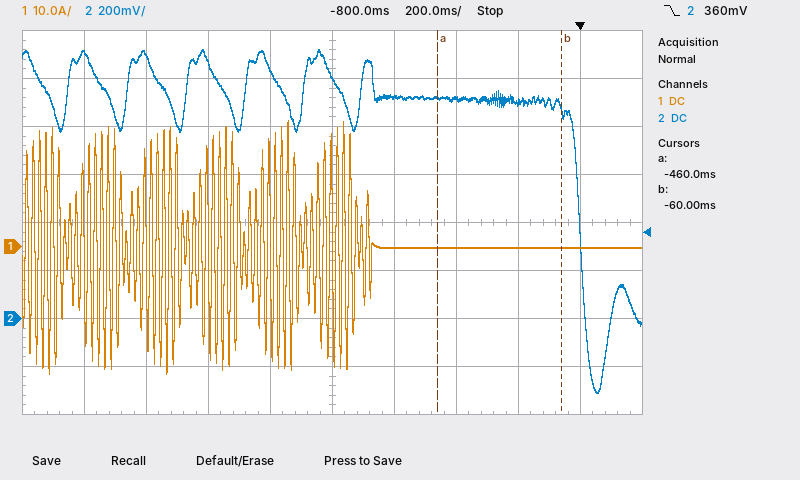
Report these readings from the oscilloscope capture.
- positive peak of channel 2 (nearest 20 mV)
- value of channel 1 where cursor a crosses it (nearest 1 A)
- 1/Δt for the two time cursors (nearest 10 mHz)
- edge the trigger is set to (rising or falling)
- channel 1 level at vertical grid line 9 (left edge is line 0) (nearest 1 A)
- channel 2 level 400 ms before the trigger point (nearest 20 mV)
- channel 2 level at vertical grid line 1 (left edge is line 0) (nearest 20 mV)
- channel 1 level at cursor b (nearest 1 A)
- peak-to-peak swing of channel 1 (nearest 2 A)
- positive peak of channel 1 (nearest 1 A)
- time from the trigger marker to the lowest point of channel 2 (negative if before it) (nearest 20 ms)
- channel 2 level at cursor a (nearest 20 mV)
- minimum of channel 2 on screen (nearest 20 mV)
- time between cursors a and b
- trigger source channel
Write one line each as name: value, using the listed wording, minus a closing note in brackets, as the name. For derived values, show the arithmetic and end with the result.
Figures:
positive peak of channel 2: 1.12 V
value of channel 1 where cursor a crosses it: 0 A
1/Δt for the two time cursors: 1 / 400 ms ≈ 2.50 Hz
edge the trigger is set to: falling
channel 1 level at vertical grid line 9 (left edge is line 0): 0 A
channel 2 level 400 ms before the trigger point: 920 mV
channel 2 level at vertical grid line 1 (left edge is line 0): 1.10 V
channel 1 level at cursor b: 0 A
peak-to-peak swing of channel 1: 52 A
positive peak of channel 1: 26 A
time from the trigger marker to the lowest point of channel 2 (negative if before it): +60 ms
channel 2 level at cursor a: 920 mV
minimum of channel 2 on screen: -300 mV
time between cursors a and b: -60 ms − (-460 ms) = 400 ms
trigger source channel: channel 2
